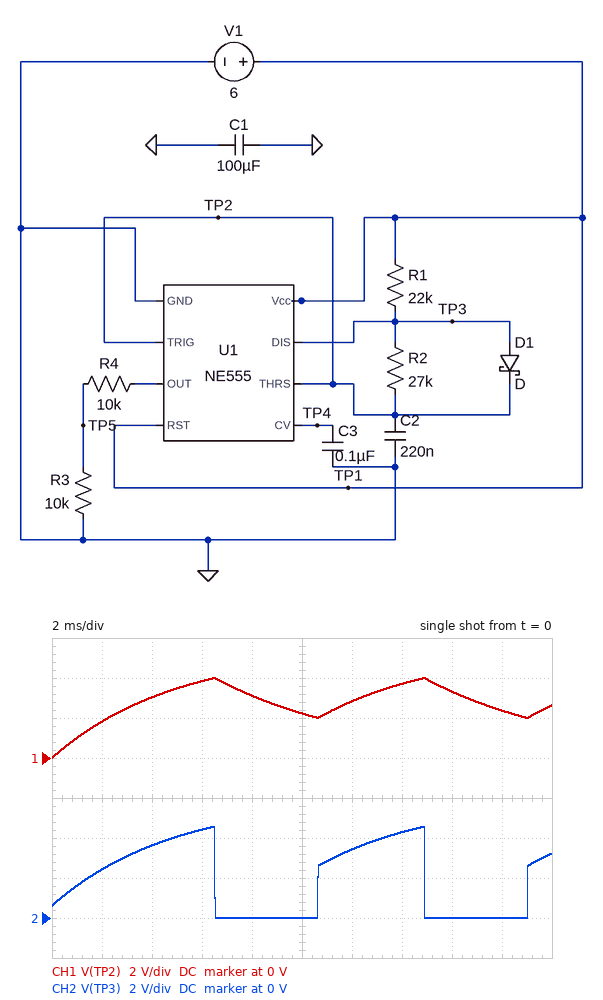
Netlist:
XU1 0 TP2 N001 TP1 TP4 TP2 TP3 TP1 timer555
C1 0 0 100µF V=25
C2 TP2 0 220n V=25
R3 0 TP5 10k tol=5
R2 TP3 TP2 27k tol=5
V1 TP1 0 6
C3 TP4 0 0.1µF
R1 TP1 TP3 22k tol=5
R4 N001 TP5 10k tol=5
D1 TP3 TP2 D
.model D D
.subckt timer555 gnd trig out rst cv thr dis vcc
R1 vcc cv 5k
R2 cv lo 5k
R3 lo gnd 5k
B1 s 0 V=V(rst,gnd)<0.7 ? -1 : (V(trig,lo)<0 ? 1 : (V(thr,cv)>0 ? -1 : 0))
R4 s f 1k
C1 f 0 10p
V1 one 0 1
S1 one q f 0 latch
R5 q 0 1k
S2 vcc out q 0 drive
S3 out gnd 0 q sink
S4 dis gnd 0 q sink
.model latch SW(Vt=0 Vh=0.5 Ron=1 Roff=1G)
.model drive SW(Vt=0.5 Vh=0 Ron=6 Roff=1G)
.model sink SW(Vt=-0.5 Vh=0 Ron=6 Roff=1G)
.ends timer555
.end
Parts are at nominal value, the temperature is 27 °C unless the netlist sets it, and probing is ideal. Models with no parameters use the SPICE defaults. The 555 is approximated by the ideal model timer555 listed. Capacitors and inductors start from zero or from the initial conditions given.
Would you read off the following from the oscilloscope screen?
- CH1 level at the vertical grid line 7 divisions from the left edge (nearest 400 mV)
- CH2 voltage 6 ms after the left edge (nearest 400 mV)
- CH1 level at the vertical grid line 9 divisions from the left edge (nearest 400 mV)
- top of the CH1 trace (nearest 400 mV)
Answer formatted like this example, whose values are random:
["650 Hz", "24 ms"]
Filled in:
["3.6 V", "4.4 V", "2.4 V", "4.0 V"]
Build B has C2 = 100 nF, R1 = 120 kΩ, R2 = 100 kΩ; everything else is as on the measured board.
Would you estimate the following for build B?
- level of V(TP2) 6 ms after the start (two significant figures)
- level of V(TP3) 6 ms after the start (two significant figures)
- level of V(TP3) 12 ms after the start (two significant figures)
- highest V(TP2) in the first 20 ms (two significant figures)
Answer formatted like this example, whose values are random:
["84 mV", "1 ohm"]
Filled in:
["2.1 V", "2.7 V", "4.0 V", "4.0 V"]
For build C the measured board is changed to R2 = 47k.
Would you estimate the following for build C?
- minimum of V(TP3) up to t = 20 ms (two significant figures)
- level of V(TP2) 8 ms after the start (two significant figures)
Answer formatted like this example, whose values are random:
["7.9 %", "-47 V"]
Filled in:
["1.9 mV", "3.5 V"]
